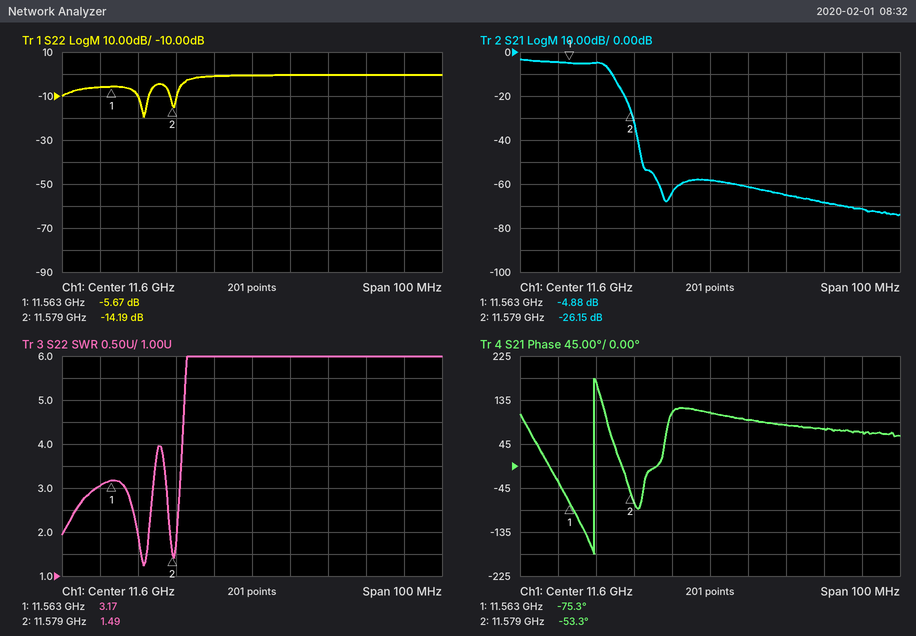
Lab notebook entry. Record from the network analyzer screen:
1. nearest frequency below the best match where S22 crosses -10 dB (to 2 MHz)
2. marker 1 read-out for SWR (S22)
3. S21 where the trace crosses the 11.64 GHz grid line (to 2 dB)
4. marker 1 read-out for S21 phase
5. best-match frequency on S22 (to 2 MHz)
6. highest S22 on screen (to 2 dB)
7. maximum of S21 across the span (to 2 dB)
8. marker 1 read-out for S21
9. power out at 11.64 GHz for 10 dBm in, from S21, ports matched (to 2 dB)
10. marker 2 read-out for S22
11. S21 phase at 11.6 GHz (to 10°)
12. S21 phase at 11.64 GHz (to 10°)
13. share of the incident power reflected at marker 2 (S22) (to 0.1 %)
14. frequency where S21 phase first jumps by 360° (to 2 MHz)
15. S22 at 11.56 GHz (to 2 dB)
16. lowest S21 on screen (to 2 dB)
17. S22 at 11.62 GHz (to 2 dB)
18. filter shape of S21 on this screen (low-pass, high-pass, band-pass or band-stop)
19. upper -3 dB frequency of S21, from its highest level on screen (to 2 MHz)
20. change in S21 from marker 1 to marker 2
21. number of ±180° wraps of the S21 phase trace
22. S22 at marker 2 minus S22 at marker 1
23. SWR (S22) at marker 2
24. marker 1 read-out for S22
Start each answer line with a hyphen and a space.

- 11.570 GHz
- 3.17
- -72 dB
- -75.3°
- 11.572 GHz
- 0 dB
- -4 dB
- -4.88 dB
- -62 dBm
- -14.19 dB
- 110°
- 70°
- 3.8 %
- 11.570 GHz
- -6 dB
- -74 dB
- 0 dB
- low-pass
- 11.572 GHz
- -21.27 dB
- 1
- -8.52 dB
- 1.49
- -5.67 dB
